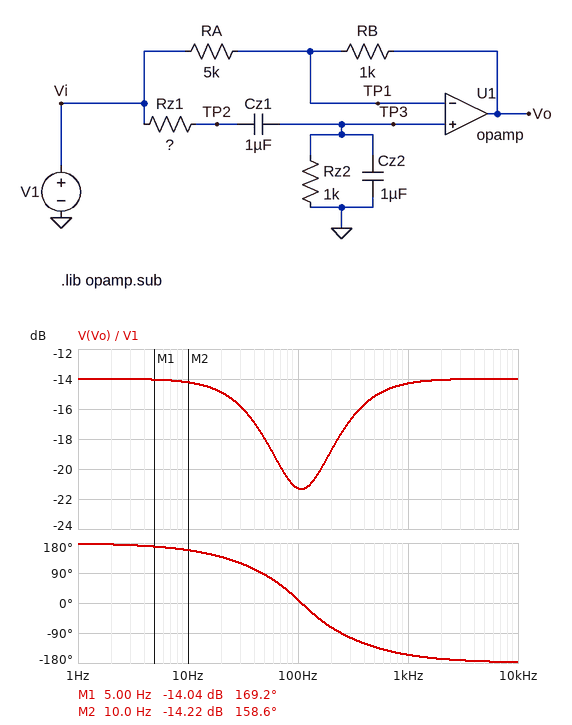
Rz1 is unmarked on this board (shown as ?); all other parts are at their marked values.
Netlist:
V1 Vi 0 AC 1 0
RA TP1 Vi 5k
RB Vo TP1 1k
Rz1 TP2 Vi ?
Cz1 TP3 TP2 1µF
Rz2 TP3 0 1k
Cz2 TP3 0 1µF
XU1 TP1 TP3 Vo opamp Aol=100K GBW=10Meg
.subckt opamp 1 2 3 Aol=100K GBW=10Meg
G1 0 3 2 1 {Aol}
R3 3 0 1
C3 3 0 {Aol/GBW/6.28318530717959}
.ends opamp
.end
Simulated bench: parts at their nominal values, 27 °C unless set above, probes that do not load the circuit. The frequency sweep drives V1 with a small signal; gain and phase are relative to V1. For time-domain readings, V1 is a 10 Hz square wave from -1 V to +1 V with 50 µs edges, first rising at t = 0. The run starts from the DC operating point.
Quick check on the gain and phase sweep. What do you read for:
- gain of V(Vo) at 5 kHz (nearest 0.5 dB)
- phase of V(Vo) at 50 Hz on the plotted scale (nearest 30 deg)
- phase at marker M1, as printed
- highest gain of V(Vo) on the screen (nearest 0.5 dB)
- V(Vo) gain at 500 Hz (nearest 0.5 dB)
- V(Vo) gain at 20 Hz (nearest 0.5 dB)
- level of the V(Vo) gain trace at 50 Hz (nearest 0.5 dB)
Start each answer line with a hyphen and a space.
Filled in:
- -14.0 dB
- 90 deg
- 169.2 deg
- -14.0 dB
- -15.0 dB
- -15.0 dB
- -18.0 dB
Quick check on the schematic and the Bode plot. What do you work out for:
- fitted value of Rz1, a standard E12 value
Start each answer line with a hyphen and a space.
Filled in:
- 2.2 kΩ
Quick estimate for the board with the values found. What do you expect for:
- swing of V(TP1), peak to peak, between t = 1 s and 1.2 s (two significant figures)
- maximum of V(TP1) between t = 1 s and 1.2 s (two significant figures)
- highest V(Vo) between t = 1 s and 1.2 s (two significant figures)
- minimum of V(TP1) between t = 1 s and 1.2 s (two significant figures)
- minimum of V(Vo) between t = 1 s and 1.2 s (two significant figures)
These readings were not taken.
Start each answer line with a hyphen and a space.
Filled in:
- 780 mV
- 390 mV
- 270 mV
- -390 mV
- -270 mV
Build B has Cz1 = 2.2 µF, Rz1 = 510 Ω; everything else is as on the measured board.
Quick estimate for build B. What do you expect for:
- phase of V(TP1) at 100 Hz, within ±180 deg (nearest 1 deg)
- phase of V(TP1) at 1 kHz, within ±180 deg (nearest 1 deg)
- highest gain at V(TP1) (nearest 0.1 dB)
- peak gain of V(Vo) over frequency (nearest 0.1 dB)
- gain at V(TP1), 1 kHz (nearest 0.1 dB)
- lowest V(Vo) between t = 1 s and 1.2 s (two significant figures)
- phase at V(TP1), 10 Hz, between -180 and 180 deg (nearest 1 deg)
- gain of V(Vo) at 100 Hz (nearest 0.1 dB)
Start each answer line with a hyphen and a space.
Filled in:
- 12 deg
- -58 deg
- -5.9 dB
- -7.7 dB
- -11.4 dB
- -880 mV
- 75 deg
- -7.9 dB
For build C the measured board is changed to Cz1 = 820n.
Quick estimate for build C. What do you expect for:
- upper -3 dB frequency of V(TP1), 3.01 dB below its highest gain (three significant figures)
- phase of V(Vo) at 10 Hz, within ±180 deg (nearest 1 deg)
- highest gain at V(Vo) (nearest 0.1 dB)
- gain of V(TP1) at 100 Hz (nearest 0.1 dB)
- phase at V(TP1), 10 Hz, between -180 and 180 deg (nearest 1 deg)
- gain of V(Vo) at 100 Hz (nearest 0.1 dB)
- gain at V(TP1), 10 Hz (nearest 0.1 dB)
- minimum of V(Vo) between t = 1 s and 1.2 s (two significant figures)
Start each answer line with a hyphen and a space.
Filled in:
- 359 Hz
- 162 deg
- -14.0 dB
- -13.0 dB
- 77 deg
- -22.5 dB
- -25.9 dB
- -240 mV
